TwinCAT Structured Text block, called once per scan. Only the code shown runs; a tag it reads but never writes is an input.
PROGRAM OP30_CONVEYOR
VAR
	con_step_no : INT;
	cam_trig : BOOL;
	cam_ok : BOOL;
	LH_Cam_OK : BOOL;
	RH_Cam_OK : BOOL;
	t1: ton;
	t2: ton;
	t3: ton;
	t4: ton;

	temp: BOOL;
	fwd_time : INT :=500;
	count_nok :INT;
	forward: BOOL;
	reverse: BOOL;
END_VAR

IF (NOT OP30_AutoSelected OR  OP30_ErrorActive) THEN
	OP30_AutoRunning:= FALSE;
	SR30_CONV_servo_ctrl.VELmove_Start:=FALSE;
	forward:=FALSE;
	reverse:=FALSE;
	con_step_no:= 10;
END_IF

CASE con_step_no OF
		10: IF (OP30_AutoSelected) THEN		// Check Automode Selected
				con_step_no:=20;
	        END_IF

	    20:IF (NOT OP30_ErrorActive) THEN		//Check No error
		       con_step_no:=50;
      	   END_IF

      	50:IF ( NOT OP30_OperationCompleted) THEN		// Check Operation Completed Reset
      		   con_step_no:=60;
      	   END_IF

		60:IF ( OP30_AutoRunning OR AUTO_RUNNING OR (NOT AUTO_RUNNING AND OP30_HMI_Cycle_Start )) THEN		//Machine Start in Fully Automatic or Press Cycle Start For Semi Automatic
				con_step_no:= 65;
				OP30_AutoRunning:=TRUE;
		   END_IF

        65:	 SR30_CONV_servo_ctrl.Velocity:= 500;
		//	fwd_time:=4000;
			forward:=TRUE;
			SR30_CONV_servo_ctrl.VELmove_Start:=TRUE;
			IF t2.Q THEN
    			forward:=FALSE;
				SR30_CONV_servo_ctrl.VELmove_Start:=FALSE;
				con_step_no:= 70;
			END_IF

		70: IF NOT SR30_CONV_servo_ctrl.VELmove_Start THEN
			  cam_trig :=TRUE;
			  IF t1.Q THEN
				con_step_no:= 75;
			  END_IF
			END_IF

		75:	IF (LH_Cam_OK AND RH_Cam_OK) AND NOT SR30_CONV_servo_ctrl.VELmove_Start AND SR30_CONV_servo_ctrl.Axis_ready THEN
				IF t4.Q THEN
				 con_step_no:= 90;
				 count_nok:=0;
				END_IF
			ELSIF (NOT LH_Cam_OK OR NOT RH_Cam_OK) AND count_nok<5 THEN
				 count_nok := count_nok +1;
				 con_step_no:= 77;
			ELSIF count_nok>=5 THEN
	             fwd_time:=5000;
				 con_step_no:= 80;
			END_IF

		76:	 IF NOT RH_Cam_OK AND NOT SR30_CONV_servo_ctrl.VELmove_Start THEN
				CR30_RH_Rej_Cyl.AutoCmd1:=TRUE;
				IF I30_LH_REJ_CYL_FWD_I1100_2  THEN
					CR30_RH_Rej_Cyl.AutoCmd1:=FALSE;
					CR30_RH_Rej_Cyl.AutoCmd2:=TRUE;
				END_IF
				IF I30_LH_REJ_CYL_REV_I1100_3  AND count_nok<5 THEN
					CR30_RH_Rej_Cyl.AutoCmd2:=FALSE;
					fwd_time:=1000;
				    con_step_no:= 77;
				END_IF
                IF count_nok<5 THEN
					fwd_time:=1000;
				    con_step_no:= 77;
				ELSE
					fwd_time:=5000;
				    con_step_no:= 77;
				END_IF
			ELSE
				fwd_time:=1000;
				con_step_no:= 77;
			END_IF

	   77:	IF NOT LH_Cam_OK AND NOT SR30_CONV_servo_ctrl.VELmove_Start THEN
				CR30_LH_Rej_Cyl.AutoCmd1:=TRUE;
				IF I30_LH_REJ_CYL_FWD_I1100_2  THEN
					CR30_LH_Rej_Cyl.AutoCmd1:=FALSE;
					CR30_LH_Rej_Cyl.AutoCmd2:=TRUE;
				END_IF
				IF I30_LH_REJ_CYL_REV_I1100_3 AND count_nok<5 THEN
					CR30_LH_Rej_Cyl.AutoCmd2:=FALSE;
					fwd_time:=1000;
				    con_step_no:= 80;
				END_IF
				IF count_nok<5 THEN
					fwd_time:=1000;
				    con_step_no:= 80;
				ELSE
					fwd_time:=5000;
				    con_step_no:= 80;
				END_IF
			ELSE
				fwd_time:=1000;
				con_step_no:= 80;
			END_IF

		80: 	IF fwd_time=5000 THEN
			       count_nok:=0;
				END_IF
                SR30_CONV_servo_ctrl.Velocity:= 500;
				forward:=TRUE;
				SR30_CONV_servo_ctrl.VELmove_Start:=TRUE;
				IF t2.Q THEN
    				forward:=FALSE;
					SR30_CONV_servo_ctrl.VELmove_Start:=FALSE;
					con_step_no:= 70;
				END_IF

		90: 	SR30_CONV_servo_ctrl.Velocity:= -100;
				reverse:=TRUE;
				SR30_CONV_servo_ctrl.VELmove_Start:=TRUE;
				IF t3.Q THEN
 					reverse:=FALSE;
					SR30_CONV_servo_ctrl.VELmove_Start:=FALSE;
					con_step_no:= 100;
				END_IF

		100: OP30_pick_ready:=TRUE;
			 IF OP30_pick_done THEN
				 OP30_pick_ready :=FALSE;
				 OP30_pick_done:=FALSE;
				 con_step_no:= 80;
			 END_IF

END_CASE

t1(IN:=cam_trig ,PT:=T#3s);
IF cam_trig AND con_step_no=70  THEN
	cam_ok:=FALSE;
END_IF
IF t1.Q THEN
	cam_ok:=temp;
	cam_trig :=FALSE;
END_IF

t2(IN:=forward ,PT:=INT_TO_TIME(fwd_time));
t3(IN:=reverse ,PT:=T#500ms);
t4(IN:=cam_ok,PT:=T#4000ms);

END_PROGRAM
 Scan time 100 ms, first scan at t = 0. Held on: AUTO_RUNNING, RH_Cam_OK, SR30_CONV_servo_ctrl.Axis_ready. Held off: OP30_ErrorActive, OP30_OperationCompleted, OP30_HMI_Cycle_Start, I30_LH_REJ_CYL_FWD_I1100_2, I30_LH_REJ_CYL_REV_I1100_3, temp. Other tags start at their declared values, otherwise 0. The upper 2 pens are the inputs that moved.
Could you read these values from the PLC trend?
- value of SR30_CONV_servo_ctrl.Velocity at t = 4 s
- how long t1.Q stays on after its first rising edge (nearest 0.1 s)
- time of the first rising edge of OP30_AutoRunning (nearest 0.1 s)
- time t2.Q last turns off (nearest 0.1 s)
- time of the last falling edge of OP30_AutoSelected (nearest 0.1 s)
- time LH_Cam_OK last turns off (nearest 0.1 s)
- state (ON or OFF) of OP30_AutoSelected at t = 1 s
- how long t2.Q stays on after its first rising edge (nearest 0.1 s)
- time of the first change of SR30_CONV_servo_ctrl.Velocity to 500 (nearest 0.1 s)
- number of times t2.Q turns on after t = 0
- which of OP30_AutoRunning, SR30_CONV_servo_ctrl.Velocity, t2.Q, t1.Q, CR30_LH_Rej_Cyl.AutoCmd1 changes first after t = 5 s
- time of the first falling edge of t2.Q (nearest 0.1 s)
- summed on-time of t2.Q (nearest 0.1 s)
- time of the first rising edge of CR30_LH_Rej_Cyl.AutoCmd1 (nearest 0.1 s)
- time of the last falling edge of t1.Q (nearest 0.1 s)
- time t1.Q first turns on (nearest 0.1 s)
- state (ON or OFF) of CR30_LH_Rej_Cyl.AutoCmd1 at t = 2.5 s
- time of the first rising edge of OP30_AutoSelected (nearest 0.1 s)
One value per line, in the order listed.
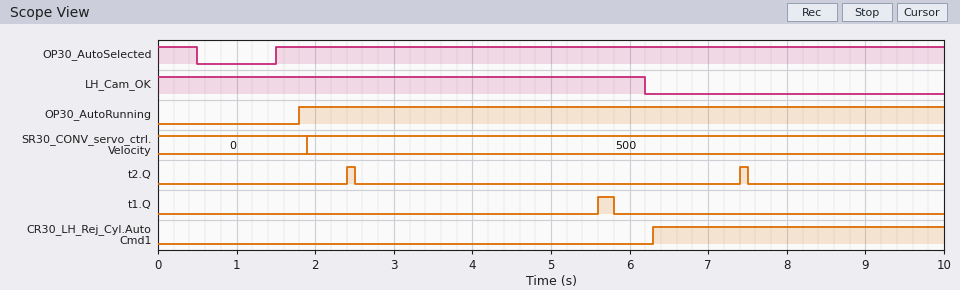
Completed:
500
0.2 s
1.8 s
7.5 s
0.5 s
6.2 s
OFF
0.1 s
1.9 s
2
t1.Q
2.5 s
0.2 s
6.3 s
5.8 s
5.6 s
OFF
1.5 s
